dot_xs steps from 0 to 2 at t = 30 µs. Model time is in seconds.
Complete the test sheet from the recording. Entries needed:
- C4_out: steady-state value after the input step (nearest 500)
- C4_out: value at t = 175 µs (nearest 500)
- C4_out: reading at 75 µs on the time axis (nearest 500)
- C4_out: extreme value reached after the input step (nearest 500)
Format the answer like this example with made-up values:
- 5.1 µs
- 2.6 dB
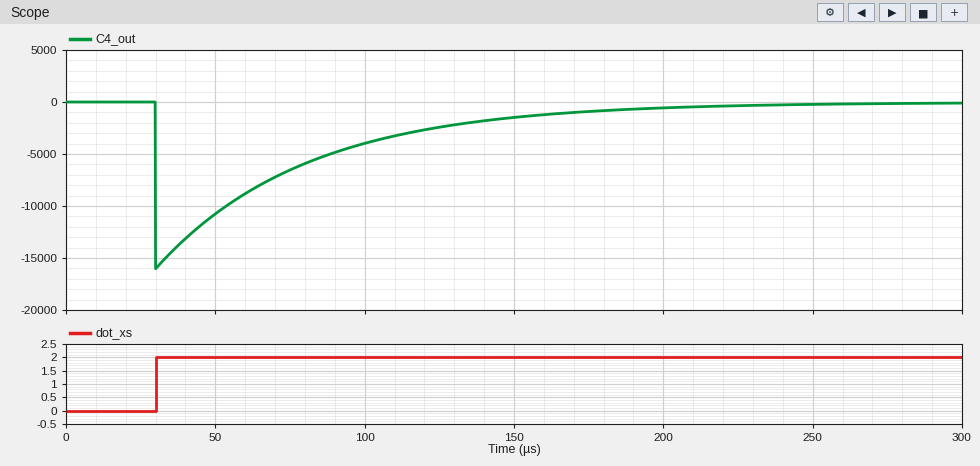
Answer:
- 0
- -1000
- -6500
- -16000
